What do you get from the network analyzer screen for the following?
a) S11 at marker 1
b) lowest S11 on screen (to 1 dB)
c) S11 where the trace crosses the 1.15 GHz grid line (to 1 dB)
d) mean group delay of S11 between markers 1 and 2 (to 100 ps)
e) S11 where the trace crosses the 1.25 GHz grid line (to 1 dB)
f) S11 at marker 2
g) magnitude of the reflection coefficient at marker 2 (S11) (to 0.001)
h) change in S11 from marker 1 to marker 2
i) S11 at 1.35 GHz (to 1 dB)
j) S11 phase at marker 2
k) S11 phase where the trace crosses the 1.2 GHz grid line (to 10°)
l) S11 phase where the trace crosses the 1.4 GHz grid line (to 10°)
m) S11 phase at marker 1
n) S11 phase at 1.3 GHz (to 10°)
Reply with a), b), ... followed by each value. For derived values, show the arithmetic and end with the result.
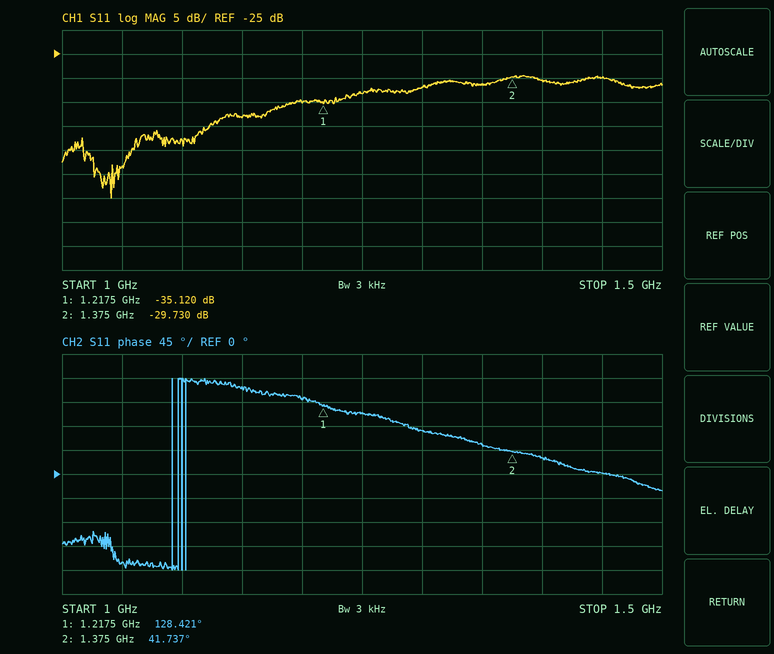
a) -35.120 dB
b) -55 dB
c) -38 dB
d) −(41.737° − (128.421°))/(360° × 157.5 MHz) ≈ 1.5 ns
e) -33 dB
f) -29.730 dB
g) 10^(-29.73/20) ≈ 0.033
h) -29.73 − (-35.12) = 5.390 dB
i) -31 dB
j) 41.737°
k) 140°
l) 30°
m) 128.421°
n) 80°
